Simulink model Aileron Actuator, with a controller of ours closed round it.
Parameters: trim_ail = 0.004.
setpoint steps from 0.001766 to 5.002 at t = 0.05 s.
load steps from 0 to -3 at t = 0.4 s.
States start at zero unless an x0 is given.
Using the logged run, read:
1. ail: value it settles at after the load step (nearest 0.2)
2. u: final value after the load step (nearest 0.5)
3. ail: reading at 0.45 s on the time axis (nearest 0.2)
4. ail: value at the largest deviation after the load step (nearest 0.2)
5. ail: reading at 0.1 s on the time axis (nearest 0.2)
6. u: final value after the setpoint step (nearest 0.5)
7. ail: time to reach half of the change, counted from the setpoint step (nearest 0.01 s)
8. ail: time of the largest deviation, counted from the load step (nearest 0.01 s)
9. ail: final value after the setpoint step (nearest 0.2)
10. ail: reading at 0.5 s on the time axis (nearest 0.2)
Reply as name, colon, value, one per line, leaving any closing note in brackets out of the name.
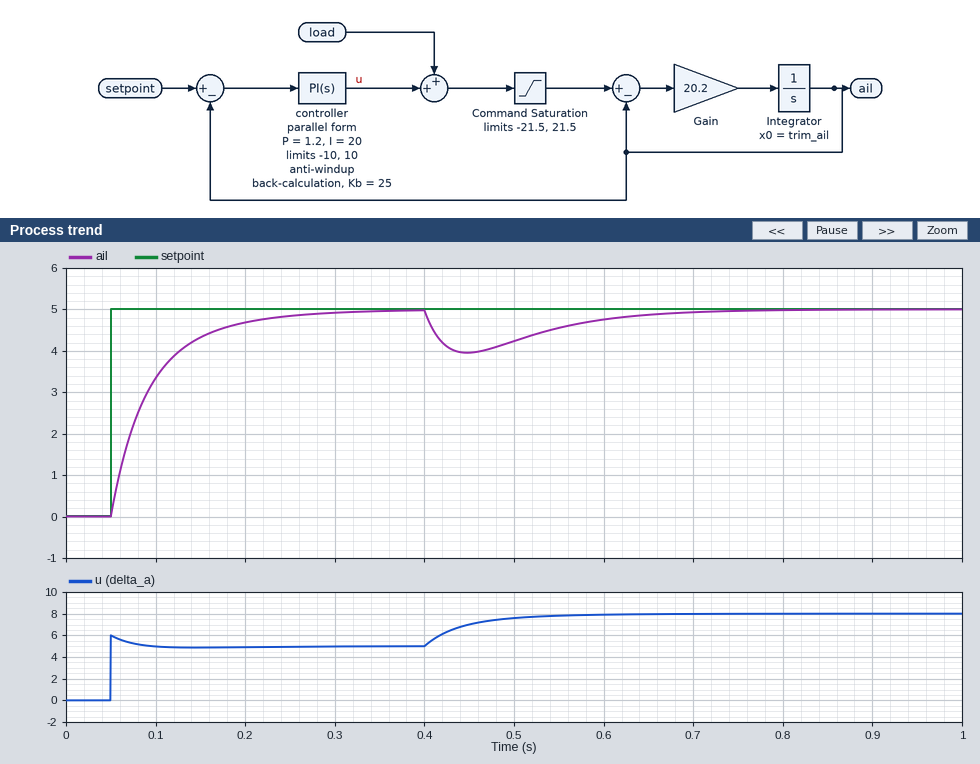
ail: value it settles at after the load step: 5.0
u: final value after the load step: 8.0
ail: reading at 0.45 s on the time axis: 4.0
ail: value at the largest deviation after the load step: 4.0
ail: reading at 0.1 s on the time axis: 3.4
u: final value after the setpoint step: 5.0
ail: time to reach half of the change, counted from the setpoint step: 0.03 s
ail: time of the largest deviation, counted from the load step: 0.05 s
ail: final value after the setpoint step: 5.0
ail: reading at 0.5 s on the time axis: 4.2
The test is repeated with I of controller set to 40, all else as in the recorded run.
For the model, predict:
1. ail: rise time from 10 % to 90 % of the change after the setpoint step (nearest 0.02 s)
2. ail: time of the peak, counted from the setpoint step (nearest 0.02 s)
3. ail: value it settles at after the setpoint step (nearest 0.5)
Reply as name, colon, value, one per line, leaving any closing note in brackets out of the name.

ail: rise time from 10 % to 90 % of the change after the setpoint step: 0.06 s
ail: time of the peak, counted from the setpoint step: 0.12 s
ail: value it settles at after the setpoint step: 5.0
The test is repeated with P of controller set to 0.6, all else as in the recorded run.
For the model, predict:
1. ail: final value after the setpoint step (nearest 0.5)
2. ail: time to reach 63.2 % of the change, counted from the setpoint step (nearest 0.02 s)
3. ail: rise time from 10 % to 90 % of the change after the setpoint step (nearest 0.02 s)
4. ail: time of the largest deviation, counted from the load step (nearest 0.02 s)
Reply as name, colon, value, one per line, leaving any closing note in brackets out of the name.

ail: final value after the setpoint step: 5.0
ail: time to reach 63.2 % of the change, counted from the setpoint step: 0.06 s
ail: rise time from 10 % to 90 % of the change after the setpoint step: 0.10 s
ail: time of the largest deviation, counted from the load step: 0.06 s
